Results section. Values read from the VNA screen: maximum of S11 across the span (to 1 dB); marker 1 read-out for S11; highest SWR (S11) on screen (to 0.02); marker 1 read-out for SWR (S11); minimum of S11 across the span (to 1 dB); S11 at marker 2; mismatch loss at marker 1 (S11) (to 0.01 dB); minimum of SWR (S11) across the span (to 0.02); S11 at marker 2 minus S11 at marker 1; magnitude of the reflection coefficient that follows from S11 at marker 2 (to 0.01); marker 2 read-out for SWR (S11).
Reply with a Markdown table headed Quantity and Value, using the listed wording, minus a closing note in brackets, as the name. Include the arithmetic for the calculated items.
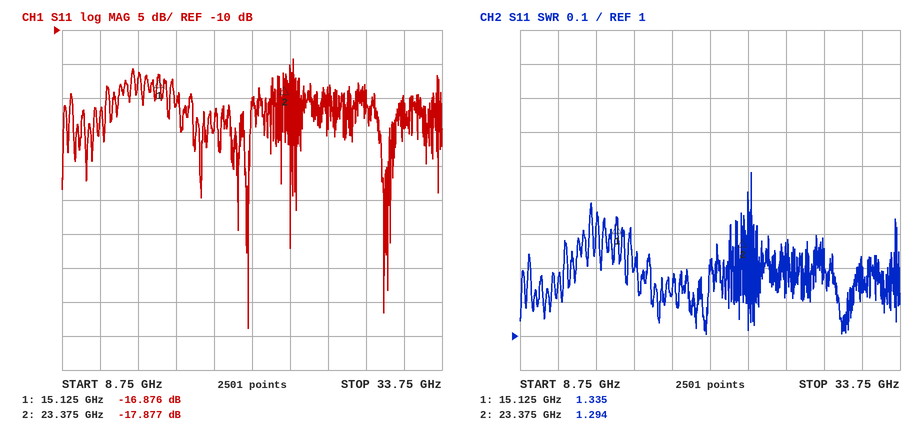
| Quantity | Value |
|---|---|
| maximum of S11 across the span | -14 dB |
| marker 1 read-out for S11 | -16.876 dB |
| highest SWR (S11) on screen | 1.48 |
| marker 1 read-out for SWR | 1.335 |
| minimum of S11 across the span | -54 dB |
| S11 at marker 2 | -17.877 dB |
| mismatch loss at marker 1 (S11) | −10 log10(1 − 10^(-16.876/10)) ≈ 0.09 dB |
| minimum of SWR (S11) across the span | 1.00 |
| S11 at marker 2 minus S11 at marker 1 | -17.877 − (-16.876) = -1.001 dB |
| magnitude of the reflection coefficient that follows from S11 at marker 2 | 10^(-17.877/20) ≈ 0.13 |
| marker 2 read-out for SWR | 1.294 |
